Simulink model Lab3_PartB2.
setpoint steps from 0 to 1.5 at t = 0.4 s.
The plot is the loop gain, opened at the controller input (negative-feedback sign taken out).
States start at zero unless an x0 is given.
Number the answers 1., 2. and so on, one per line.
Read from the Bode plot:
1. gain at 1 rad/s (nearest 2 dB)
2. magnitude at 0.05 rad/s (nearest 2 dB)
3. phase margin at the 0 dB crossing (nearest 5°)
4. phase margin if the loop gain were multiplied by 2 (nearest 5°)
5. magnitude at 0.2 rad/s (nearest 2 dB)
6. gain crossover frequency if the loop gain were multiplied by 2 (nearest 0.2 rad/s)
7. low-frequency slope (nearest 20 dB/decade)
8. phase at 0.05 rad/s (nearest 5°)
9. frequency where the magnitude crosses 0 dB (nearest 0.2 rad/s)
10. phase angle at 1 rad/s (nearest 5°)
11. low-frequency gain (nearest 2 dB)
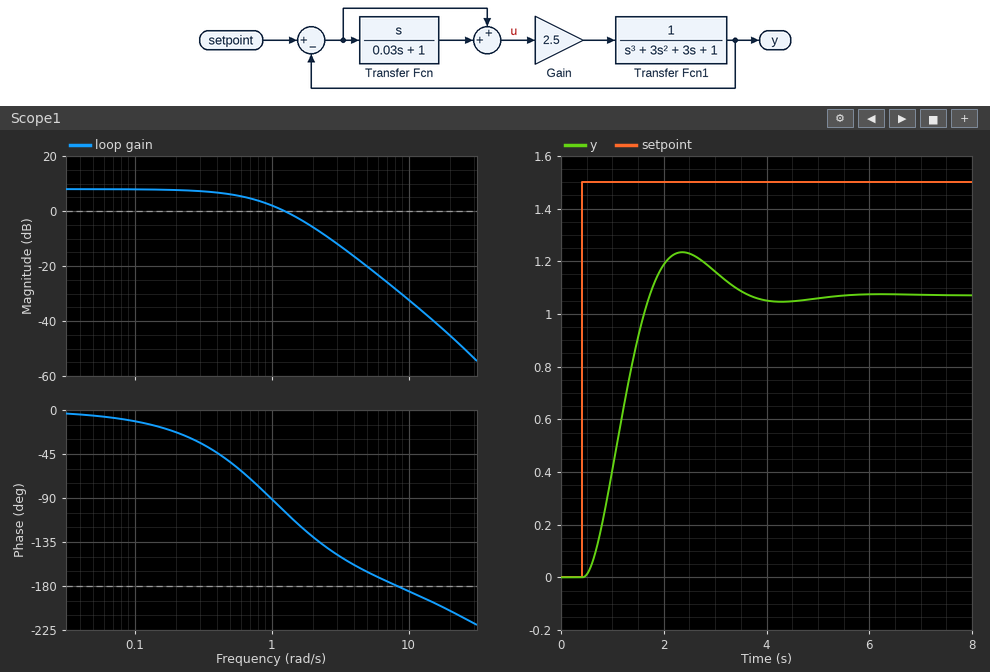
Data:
1. 2 dB
2. 8 dB
3. 75°
4. 50°
5. 8 dB
6. 2.0 rad/s
7. 0 dB/decade
8. -5°
9. 1.2 rad/s
10. -90°
11. 8 dB
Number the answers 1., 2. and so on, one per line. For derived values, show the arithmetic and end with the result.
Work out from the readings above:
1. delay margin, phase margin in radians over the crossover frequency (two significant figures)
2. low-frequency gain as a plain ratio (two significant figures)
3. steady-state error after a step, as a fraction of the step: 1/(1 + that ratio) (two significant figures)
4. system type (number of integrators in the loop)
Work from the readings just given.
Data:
1. 75 × π / 180 / 1.2 = 1.1 s
2. 10^(8 / 20) = 2.5
3. 1 / (1 + 2.5) = 0.29
4. 0
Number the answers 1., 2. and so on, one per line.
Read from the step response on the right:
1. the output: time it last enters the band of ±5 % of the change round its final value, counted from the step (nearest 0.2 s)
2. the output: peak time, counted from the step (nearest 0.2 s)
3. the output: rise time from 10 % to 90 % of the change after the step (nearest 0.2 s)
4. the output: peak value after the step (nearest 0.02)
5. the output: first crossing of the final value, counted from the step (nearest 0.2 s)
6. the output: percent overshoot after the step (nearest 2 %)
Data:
1. 2.8 s
2. 2.0 s
3. 0.8 s
4. 1.24
5. 1.4 s
6. 16 %
